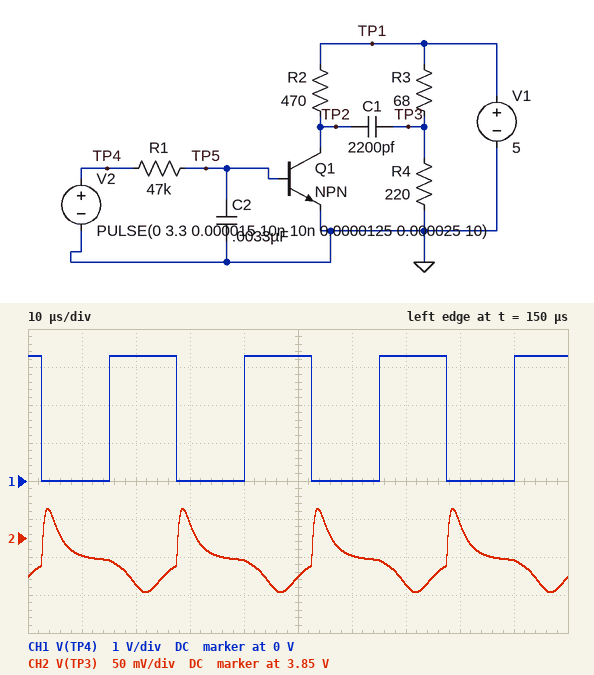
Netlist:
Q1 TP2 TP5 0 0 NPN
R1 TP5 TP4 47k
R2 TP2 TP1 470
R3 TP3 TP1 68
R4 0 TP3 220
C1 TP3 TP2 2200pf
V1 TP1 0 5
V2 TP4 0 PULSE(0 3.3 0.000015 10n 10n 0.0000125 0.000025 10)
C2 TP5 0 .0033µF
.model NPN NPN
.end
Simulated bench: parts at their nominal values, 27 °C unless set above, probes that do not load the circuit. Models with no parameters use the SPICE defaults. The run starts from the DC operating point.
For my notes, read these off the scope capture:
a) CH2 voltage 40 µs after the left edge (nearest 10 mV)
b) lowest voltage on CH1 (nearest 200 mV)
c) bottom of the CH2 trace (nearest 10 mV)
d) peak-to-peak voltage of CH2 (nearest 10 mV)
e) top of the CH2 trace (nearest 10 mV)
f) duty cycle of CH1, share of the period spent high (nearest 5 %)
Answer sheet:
3.82 V
0 V
3.78 V
110 mV
3.89 V
50 %
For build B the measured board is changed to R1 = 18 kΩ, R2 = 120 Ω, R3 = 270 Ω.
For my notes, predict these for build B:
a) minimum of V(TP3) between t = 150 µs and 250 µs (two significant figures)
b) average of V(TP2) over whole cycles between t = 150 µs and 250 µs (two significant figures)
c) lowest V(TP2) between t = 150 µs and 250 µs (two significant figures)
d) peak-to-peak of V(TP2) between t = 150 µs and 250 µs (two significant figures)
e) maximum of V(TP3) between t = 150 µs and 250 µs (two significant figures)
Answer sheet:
2.1 V
4.4 V
3.4 V
1.6 V
2.5 V
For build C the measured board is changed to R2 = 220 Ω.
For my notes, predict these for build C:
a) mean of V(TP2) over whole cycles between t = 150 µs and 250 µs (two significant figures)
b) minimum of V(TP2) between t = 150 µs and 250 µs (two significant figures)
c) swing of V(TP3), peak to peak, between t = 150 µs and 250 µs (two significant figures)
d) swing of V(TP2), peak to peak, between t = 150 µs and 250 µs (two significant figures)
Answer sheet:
4.6 V
3.9 V
65 mV
1.1 V
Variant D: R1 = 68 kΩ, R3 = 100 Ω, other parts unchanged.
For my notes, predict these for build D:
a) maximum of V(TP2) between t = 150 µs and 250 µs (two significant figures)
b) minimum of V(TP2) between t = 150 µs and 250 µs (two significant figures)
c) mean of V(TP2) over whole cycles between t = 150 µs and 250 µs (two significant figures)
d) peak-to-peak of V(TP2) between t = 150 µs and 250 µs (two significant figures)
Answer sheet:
4.9 V
3.5 V
4.4 V
1.4 V
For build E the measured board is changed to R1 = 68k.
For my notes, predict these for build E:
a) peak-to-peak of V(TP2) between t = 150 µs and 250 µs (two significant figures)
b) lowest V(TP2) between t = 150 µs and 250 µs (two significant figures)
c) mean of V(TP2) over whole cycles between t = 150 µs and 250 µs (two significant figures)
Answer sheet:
1.4 V
3.5 V
4.4 V
